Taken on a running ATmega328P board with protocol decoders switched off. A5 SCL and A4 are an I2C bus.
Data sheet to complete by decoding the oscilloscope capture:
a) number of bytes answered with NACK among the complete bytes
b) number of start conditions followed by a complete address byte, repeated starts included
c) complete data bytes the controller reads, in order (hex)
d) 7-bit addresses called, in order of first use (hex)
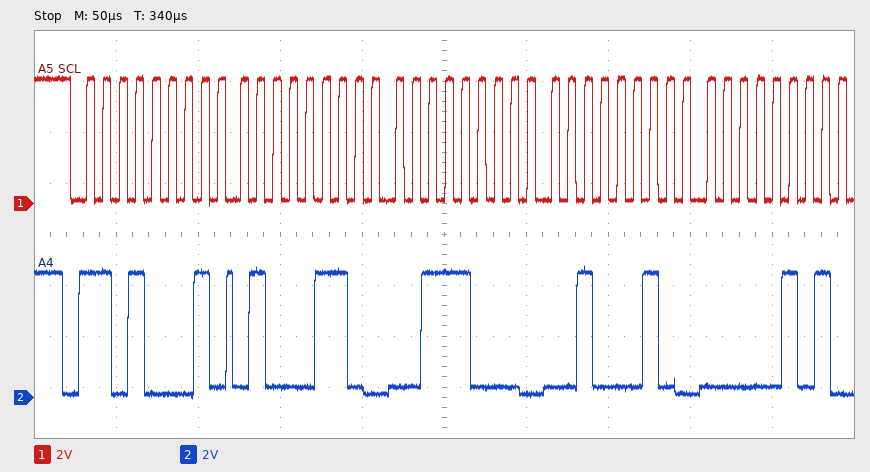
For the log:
0
1
46 38 22 05
0x68
